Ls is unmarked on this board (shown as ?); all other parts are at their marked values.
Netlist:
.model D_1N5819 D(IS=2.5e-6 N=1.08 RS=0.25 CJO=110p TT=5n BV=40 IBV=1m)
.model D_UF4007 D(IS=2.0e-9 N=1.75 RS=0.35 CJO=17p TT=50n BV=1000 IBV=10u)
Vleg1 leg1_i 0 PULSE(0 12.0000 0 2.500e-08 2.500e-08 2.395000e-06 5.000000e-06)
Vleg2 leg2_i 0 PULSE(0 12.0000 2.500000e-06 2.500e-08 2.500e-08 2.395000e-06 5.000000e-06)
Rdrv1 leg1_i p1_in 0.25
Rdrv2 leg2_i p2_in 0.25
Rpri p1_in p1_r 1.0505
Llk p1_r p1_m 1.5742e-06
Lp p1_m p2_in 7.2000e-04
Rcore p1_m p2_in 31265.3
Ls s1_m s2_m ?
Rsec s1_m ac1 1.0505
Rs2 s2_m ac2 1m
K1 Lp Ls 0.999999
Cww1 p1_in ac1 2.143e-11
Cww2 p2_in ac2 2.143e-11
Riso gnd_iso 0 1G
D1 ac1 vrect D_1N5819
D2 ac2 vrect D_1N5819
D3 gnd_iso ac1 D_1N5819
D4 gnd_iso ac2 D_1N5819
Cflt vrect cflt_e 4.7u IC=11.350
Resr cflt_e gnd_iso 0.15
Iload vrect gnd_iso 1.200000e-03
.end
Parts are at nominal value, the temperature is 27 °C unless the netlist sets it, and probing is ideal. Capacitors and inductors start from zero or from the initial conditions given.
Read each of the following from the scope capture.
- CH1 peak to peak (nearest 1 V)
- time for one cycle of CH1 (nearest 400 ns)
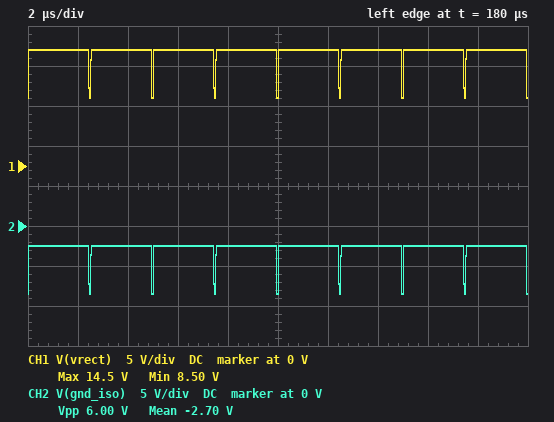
6 V
2.4 µs
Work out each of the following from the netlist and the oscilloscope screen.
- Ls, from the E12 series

1.5 mH
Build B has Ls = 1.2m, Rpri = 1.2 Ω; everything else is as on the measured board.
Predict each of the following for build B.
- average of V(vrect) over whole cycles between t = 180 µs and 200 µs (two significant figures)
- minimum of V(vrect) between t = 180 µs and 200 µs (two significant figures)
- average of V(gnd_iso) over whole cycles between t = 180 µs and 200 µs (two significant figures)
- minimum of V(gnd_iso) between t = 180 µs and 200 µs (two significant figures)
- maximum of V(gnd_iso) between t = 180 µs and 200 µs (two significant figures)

13 V
7.6 V
-1.8 V
-7.6 V
-1.6 V
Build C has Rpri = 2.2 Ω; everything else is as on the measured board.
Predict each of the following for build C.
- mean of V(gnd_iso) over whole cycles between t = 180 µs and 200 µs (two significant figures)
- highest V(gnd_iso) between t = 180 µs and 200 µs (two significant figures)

-2.6 V
-2.4 V
